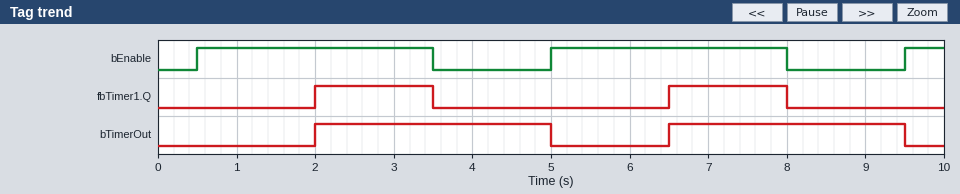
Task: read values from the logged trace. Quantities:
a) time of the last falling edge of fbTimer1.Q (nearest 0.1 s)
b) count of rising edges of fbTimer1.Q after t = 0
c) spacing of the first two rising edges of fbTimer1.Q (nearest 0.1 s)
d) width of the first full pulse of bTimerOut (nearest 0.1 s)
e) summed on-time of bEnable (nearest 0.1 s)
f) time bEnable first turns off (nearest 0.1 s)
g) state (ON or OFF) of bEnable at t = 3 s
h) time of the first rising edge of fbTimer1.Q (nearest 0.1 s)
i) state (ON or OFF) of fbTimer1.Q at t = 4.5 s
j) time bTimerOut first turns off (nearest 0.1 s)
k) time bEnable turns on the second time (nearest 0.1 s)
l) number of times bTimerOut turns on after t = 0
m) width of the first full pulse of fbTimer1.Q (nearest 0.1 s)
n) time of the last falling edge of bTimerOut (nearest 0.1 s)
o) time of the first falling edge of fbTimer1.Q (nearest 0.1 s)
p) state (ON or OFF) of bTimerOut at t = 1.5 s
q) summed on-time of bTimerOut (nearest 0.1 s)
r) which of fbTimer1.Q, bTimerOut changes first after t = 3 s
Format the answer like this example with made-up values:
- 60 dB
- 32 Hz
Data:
- 8.0 s
- 2
- 4.5 s
- 3.0 s
- 6.5 s
- 3.5 s
- ON
- 2.0 s
- OFF
- 5.0 s
- 5.0 s
- 2
- 1.5 s
- 9.5 s
- 3.5 s
- OFF
- 6.0 s
- fbTimer1.Q
